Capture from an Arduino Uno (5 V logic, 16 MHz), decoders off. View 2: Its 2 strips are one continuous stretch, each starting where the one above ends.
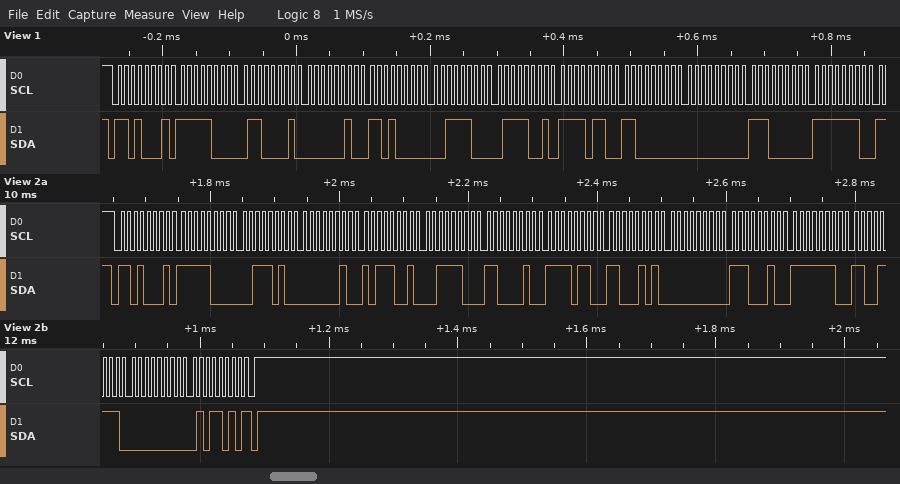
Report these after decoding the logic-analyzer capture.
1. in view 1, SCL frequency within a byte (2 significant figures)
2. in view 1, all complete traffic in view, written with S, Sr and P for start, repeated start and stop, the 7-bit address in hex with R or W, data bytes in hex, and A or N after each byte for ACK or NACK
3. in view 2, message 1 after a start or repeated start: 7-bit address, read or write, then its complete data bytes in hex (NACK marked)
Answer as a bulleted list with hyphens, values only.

- 100 kHz
- S 68R A F8 A 61 A 02 A D0 A 3C A 79 A F6 A C0 A 00 A E0 A FE A
- 0x68 read: F8 3A 02 B9 3C C2 F6 C5 00 E2 FE CF 00 5A NACK
